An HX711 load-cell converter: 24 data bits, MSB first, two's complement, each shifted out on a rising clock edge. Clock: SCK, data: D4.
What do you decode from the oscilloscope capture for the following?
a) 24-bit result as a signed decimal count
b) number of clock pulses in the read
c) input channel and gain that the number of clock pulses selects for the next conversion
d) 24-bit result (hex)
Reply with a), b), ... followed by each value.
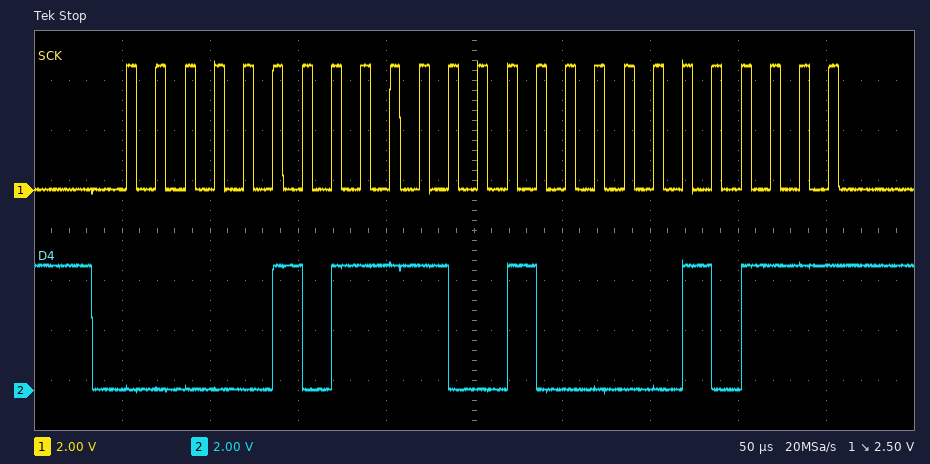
a) 386071
b) 25
c) channel A, gain 128
d) 0x05E417
